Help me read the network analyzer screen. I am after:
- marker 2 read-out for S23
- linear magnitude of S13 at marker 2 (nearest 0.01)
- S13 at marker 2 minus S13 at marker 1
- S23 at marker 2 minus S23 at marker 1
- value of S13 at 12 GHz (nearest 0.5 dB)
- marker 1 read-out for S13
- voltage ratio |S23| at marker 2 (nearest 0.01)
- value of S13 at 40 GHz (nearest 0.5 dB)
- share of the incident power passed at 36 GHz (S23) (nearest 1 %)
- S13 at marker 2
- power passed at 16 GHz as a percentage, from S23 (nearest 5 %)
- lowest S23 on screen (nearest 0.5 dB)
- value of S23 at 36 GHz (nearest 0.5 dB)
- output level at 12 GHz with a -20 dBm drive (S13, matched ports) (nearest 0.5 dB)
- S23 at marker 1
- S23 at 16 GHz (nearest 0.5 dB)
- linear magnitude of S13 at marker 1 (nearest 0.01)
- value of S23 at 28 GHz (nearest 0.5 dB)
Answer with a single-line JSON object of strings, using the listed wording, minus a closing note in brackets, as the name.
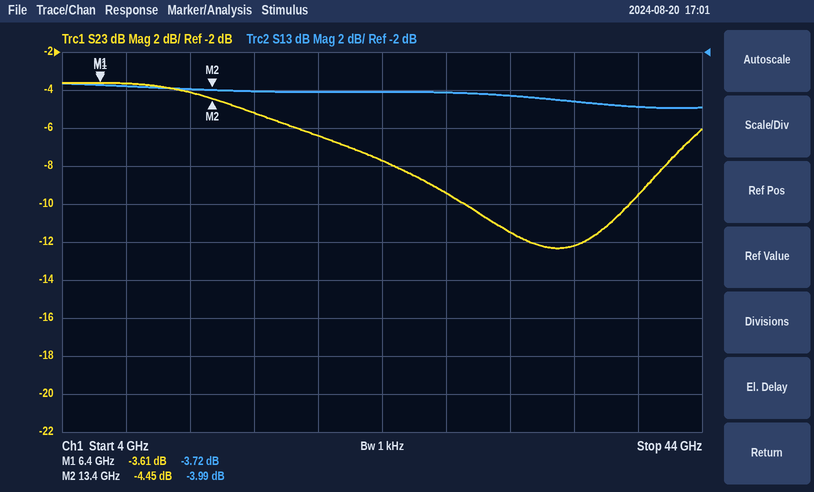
{"marker 2 read-out for S23": "-4.45 dB", "linear magnitude of S13 at marker 2": "0.63", "S13 at marker 2 minus S13 at marker 1": "-0.27 dB", "S23 at marker 2 minus S23 at marker 1": "-0.84 dB", "value of S13 at 12 GHz": "-4.0 dB", "marker 1 read-out for S13": "-3.72 dB", "voltage ratio |S23| at marker 2": "0.60", "value of S13 at 40 GHz": "-5.0 dB", "share of the incident power passed at 36 GHz (S23)": "6 %", "S13 at marker 2": "-3.99 dB", "power passed at 16 GHz as a percentage, from S23": "30 %", "lowest S23 on screen": "-12.5 dB", "value of S23 at 36 GHz": "-12.0 dB", "output level at 12 GHz with a -20 dBm drive (S13, matched ports)": "-24.0 dBm", "S23 at marker 1": "-3.61 dB", "S23 at 16 GHz": "-5.0 dB", "linear magnitude of S13 at marker 1": "0.65", "value of S23 at 28 GHz": "-9.5 dB"}
